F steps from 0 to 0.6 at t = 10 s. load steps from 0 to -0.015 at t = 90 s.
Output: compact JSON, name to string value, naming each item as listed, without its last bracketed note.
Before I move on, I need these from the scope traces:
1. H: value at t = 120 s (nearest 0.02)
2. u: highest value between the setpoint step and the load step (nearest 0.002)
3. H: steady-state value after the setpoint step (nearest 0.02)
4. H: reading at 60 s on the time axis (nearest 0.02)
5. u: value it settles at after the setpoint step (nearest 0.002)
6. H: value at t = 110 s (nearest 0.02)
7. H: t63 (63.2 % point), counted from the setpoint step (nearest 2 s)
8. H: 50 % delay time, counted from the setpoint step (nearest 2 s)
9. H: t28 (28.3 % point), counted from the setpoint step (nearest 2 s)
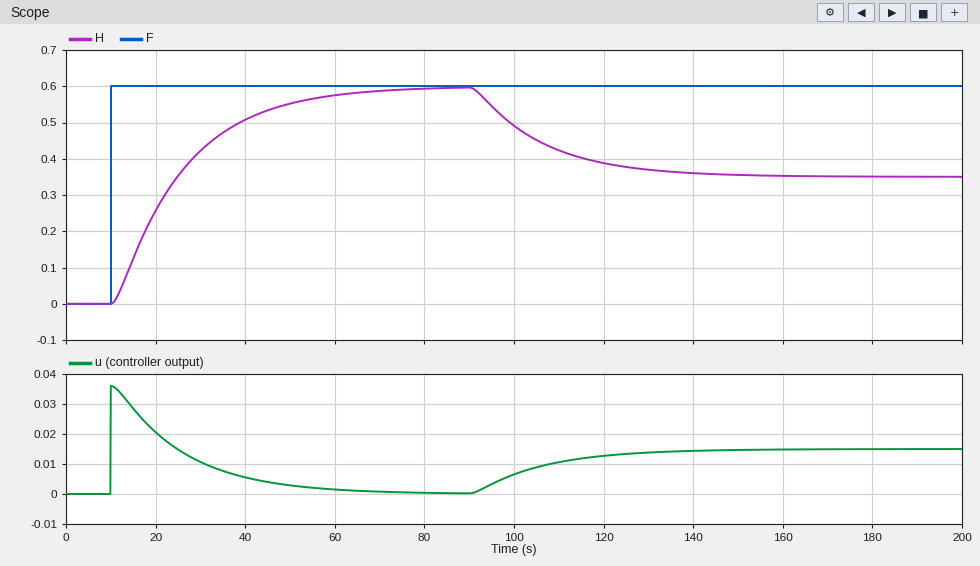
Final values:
{"H: value at t = 120 s": "0.38", "u: highest value between the setpoint step and the load step": "0.036", "H: steady-state value after the setpoint step": "0.60", "H: reading at 60 s on the time axis": "0.58", "u: value it settles at after the setpoint step": "0.000", "H: value at t = 110 s": "0.42", "H: t63 (63.2 % point), counted from the setpoint step": "16 s", "H: 50 % delay time, counted from the setpoint step": "12 s", "H: t28 (28.3 % point), counted from the setpoint step": "6 s"}
